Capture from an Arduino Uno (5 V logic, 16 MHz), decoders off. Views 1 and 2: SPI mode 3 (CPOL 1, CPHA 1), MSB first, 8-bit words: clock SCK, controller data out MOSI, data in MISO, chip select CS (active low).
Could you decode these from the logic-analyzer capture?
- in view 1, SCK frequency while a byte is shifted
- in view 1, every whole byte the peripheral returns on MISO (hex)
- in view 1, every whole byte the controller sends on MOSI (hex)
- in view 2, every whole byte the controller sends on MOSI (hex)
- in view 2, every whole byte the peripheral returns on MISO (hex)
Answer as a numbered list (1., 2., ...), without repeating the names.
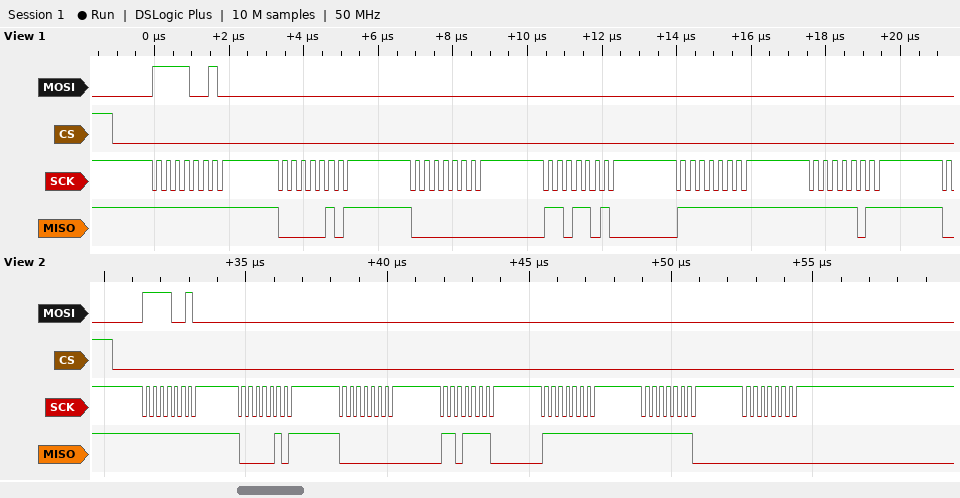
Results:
1. 4 MHz
2. FF 05 00 DA FF FB
3. F2 00 00 00 00 00
4. F2 00 00 00 00 00 00
5. FF 05 00 DE FF FE 00
